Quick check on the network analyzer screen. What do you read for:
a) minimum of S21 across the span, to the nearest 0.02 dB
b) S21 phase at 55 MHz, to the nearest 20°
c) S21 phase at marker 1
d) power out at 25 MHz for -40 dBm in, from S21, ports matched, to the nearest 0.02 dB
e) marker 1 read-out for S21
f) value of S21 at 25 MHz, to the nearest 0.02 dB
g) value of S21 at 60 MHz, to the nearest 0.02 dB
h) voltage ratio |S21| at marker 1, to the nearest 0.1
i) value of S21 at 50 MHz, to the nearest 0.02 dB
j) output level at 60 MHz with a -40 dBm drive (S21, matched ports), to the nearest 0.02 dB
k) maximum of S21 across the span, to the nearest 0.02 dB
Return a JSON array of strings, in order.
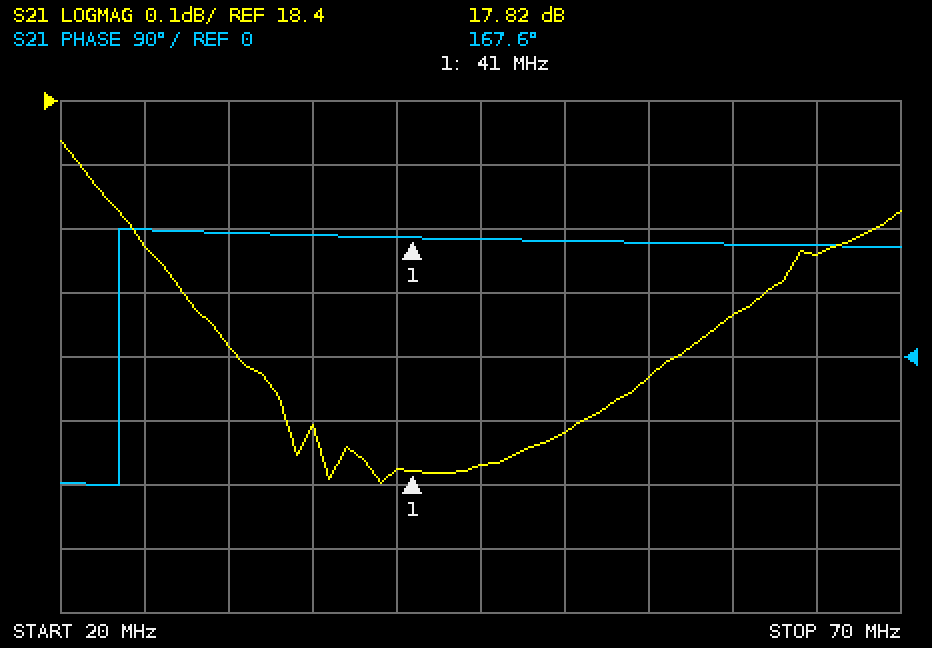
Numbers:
["17.80 dB", "160°", "167.6°", "-21.82 dBm", "17.82 dB", "18.18 dB", "18.06 dB", "7.8", "17.88 dB", "-21.94 dBm", "18.34 dB"]
